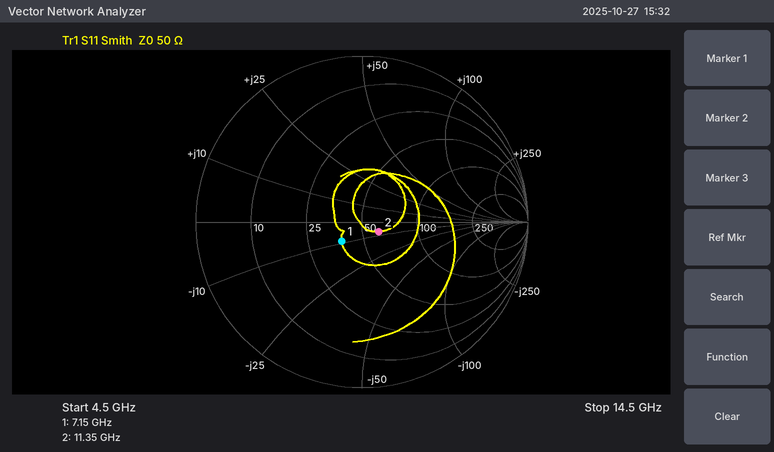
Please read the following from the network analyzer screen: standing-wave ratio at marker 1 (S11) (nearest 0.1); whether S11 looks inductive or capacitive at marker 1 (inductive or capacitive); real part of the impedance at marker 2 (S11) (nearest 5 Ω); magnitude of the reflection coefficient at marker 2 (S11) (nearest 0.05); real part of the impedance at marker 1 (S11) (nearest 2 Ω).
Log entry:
1.4
capacitive
60 Ω
0.10
38 Ω
